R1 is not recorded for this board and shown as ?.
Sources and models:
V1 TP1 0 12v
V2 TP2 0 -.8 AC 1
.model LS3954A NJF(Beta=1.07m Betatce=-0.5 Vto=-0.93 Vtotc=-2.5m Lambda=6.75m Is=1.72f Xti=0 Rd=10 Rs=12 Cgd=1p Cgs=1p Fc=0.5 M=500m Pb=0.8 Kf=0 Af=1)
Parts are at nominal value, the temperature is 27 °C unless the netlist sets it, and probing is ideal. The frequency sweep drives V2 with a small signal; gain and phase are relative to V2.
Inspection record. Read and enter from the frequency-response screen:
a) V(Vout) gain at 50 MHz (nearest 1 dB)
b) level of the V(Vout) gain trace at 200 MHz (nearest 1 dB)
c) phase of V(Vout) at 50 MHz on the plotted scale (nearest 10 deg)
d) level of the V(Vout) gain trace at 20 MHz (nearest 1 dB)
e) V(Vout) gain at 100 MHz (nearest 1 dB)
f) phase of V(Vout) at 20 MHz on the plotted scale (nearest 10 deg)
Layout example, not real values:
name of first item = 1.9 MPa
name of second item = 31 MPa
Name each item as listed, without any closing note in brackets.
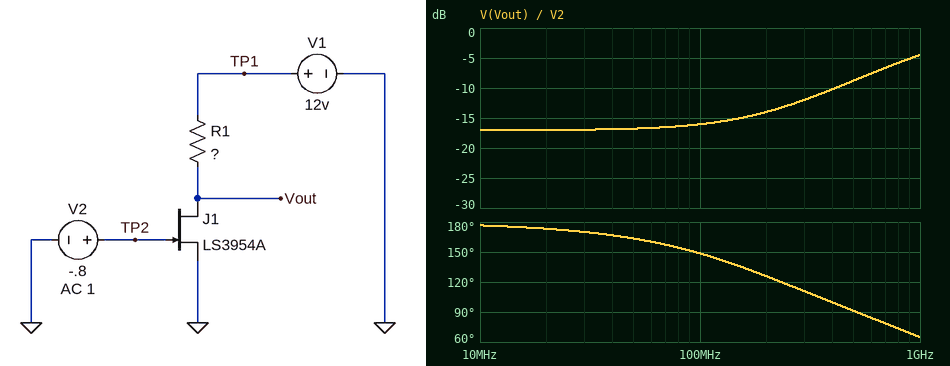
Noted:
V(Vout) gain at 50 MHz = -17 dB
level of the V(Vout) gain trace at 200 MHz = -14 dB
phase of V(Vout) at 50 MHz on the plotted scale = 160 deg
level of the V(Vout) gain trace at 20 MHz = -17 dB
V(Vout) gain at 100 MHz = -16 dB
phase of V(Vout) at 20 MHz on the plotted scale = 170 deg
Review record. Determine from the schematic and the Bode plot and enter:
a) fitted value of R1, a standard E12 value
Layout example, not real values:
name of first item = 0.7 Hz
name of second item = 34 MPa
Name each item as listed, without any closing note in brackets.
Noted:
fitted value of R1, a standard E12 value = 470 Ω
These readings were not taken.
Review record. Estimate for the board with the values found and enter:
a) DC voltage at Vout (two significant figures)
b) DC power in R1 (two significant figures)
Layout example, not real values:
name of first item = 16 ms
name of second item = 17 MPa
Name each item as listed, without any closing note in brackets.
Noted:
DC voltage at Vout = 12 V
DC power in R1 = 180 nW
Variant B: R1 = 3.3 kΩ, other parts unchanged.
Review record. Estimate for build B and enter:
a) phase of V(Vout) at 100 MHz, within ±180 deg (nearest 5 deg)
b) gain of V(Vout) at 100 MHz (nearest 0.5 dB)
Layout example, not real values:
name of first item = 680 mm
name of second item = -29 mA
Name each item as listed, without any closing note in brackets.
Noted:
phase of V(Vout) at 100 MHz, within ±180 deg = 125 deg
gain of V(Vout) at 100 MHz = 0 dB
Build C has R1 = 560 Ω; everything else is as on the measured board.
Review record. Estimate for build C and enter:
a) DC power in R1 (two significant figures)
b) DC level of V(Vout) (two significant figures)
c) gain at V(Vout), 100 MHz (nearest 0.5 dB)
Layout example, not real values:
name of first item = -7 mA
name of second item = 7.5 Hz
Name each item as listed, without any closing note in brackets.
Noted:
DC power in R1 = 210 nW
DC level of V(Vout) = 12 V
gain at V(Vout), 100 MHz = -14.5 dB
